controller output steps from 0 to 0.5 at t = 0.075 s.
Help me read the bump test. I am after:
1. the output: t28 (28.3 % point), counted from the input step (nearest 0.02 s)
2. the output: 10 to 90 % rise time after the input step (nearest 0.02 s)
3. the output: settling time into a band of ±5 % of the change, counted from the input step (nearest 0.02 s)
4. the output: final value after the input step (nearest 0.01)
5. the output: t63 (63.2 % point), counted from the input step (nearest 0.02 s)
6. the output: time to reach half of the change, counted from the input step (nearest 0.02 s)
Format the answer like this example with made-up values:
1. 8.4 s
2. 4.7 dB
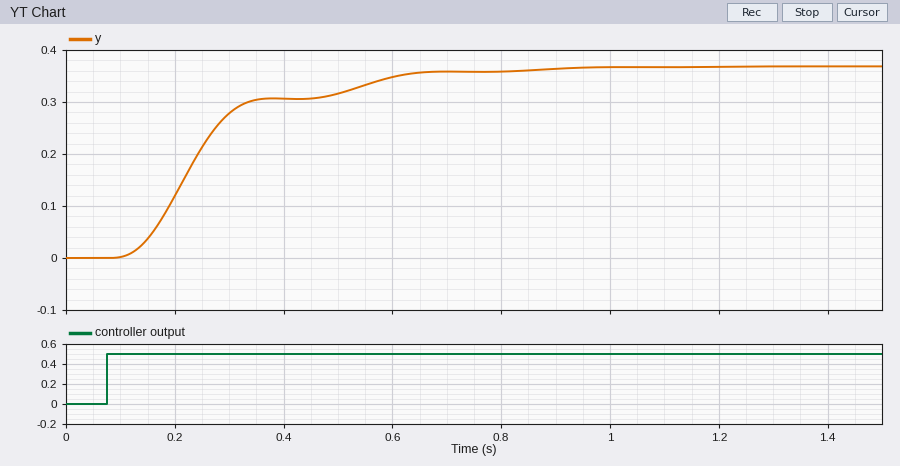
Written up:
1. 0.12 s
2. 0.40 s
3. 0.54 s
4. 0.37
5. 0.18 s
6. 0.16 s
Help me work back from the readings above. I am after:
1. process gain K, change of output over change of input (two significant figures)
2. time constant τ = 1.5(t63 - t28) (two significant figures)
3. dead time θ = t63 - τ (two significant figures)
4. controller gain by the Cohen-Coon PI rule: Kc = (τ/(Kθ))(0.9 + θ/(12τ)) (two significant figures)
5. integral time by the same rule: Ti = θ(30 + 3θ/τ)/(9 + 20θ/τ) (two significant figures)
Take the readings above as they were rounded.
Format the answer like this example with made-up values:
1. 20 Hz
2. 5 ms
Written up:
1. 0.74
2. 0.090 s
3. 0.090 s
4. 1.3
5. 0.10 s
